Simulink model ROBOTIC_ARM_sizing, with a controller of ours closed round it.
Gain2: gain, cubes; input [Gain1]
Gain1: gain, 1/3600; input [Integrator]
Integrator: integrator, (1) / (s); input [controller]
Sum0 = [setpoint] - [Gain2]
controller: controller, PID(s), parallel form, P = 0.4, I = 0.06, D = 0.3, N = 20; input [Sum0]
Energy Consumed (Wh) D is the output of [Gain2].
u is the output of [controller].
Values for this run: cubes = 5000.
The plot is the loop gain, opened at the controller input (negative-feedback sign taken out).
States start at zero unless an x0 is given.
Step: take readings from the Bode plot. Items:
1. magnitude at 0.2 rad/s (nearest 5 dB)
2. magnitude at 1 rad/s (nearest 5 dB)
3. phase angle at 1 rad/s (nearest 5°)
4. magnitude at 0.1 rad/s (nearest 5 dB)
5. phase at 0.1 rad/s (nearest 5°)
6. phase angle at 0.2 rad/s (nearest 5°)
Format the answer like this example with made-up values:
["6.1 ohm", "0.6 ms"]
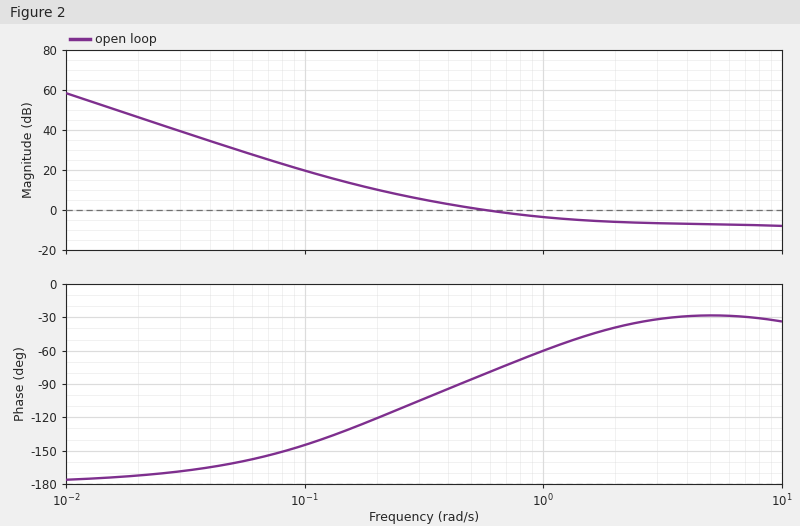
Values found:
["10 dB", "-5 dB", "-60°", "20 dB", "-145°", "-120°"]
